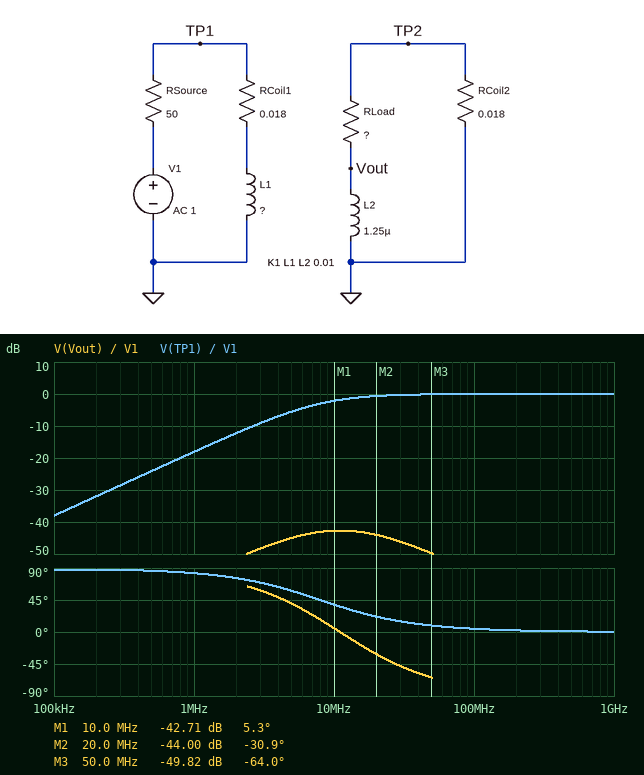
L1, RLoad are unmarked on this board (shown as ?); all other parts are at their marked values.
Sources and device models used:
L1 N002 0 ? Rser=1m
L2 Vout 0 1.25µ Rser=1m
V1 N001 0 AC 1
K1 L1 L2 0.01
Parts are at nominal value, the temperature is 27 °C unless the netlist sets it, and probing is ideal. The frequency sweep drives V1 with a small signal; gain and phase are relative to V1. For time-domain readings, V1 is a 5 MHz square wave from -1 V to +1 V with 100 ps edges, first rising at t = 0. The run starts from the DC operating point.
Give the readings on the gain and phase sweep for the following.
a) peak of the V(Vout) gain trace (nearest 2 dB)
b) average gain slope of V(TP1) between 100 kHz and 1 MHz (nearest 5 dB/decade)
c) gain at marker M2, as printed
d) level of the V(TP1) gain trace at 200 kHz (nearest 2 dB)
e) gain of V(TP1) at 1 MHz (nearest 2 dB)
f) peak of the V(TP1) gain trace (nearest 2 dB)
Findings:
-42 dB
20 dB/decade
-44.00 dB
-32 dB
-18 dB
0 dB
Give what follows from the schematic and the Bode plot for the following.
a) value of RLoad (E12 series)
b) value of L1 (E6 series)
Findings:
120 Ω
1 µH
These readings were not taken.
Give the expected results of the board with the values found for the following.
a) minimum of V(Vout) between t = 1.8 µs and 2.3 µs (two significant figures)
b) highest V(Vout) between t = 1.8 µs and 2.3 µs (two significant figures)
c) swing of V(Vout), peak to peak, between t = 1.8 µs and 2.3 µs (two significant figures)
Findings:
-11 mV
11 mV
22 mV
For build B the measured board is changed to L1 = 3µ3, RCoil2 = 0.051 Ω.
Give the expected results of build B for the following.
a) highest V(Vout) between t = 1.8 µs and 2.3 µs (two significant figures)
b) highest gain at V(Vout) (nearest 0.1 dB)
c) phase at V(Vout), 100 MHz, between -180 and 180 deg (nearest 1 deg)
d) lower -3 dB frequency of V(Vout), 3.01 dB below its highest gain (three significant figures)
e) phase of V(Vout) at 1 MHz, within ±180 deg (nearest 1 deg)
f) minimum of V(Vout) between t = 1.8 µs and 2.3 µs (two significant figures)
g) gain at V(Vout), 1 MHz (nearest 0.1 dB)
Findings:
6.9 mV
-45.5 dB
-80 deg
1.88 MHz
64 deg
-6.9 mV
-52.6 dB
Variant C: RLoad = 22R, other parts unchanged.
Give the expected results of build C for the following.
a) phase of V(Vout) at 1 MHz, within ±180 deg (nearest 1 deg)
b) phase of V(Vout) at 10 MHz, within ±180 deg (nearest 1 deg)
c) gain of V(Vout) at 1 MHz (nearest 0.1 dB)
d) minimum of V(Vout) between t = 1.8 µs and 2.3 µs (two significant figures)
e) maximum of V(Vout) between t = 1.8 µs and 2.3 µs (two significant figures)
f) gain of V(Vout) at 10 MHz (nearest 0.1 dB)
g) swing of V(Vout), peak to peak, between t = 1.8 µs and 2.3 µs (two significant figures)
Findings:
63 deg
-36 deg
-57.6 dB
-3.5 mV
3.5 mV
-52.5 dB
7.0 mV
